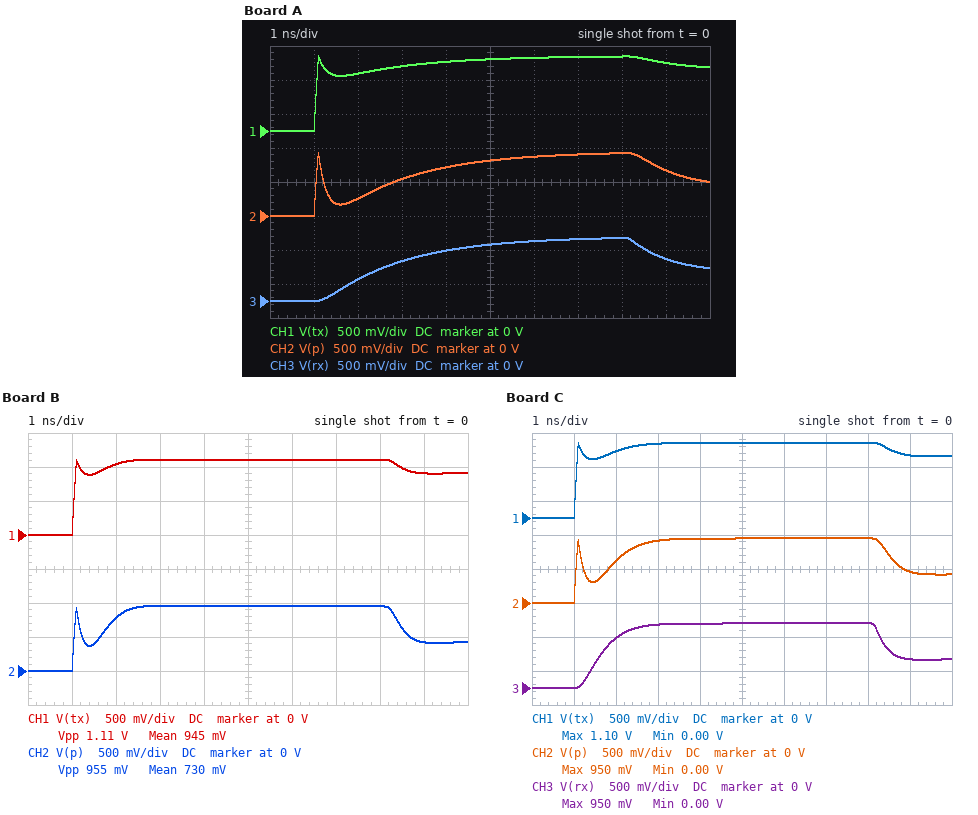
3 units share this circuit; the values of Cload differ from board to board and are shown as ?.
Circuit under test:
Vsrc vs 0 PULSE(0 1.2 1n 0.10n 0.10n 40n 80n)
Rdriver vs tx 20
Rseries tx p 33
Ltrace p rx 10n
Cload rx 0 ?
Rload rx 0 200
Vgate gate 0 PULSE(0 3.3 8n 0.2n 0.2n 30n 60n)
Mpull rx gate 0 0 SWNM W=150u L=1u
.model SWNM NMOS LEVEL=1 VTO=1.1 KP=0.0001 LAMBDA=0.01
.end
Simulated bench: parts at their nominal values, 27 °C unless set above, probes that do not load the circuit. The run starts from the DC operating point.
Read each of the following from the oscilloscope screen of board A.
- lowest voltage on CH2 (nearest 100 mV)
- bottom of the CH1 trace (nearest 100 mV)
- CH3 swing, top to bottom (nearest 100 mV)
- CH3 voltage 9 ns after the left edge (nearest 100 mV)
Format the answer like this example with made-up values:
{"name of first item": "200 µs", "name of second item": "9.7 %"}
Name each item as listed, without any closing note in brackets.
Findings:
{"lowest voltage on CH2": "0 V", "bottom of the CH1 trace": "0 V", "CH3 swing, top to bottom": "900 mV", "CH3 voltage 9 ns after the left edge": "600 mV"}
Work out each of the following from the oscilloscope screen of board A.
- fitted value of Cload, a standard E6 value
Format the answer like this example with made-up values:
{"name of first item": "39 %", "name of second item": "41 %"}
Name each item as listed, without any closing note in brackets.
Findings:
{"fitted value of Cload, a standard E6 value": "47 pF"}
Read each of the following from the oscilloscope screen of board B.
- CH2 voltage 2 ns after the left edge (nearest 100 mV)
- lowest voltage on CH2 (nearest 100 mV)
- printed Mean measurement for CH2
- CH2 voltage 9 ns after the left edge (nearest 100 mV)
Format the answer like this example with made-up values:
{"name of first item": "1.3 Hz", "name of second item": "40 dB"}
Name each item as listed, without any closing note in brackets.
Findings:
{"CH2 voltage 2 ns after the left edge": "800 mV", "lowest voltage on CH2": "0 V", "printed Mean measurement for CH2": "730 mV", "CH2 voltage 9 ns after the left edge": "400 mV"}
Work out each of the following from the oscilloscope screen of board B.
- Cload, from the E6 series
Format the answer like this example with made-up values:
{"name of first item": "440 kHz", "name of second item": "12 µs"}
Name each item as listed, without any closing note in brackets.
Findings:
{"Cload, from the E6 series": "10 pF"}
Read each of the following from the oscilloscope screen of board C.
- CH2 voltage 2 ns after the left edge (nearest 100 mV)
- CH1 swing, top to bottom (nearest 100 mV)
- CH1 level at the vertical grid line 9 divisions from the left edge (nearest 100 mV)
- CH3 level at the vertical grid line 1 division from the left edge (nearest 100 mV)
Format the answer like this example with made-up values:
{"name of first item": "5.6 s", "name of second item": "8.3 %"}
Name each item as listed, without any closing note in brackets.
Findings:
{"CH2 voltage 2 ns after the left edge": "600 mV", "CH1 swing, top to bottom": "1.1 V", "CH1 level at the vertical grid line 9 divisions from the left edge": "900 mV", "CH3 level at the vertical grid line 1 division from the left edge": "0 V"}
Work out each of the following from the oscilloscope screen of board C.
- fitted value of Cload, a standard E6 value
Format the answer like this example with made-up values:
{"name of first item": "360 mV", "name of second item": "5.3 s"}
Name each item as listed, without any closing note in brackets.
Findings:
{"fitted value of Cload, a standard E6 value": "15 pF"}
